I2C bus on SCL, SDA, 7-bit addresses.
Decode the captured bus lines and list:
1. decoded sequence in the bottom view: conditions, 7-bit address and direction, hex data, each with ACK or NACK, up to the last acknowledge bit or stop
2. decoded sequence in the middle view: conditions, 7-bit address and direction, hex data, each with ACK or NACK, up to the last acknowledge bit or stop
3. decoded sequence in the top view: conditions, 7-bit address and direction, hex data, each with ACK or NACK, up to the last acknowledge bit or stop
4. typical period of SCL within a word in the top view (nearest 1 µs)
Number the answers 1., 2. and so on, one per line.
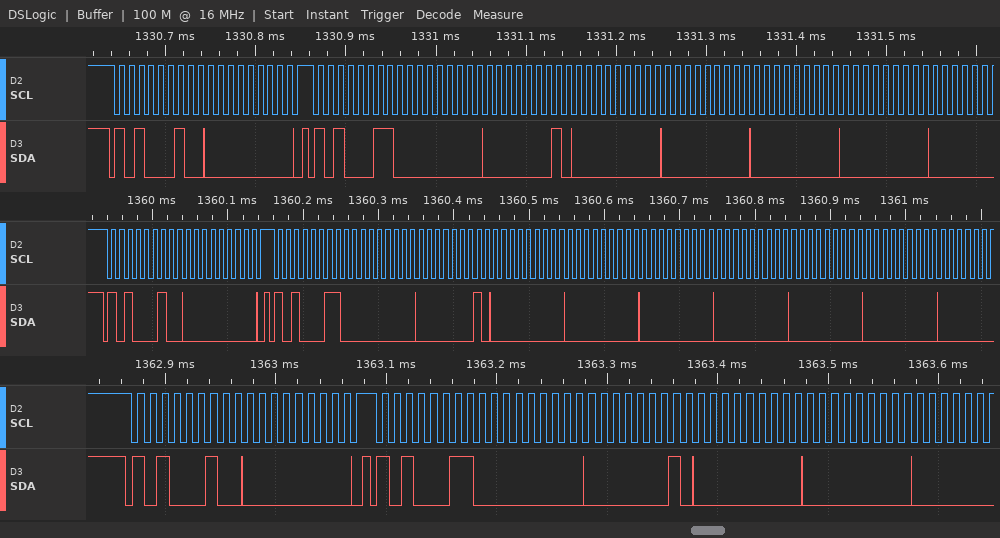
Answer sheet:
1. start, address 51 write ACK, 00 ACK, stop, start, address 51 read ACK, 00 ACK, 02 ACK, 00 ACK, 00 ACK
2. start, address 51 write ACK, 00 ACK, stop, start, address 51 read ACK, 00 ACK, 02 ACK, 00 ACK, 00 ACK, 00 ACK, 00 ACK, 00 ACK, 00 ACK
3. start, address 51 write ACK, 00 ACK, stop, start, address 51 read ACK, 00 ACK, 02 ACK, 00 ACK, 00 ACK, 00 ACK, 00 ACK
4. 11 µs
